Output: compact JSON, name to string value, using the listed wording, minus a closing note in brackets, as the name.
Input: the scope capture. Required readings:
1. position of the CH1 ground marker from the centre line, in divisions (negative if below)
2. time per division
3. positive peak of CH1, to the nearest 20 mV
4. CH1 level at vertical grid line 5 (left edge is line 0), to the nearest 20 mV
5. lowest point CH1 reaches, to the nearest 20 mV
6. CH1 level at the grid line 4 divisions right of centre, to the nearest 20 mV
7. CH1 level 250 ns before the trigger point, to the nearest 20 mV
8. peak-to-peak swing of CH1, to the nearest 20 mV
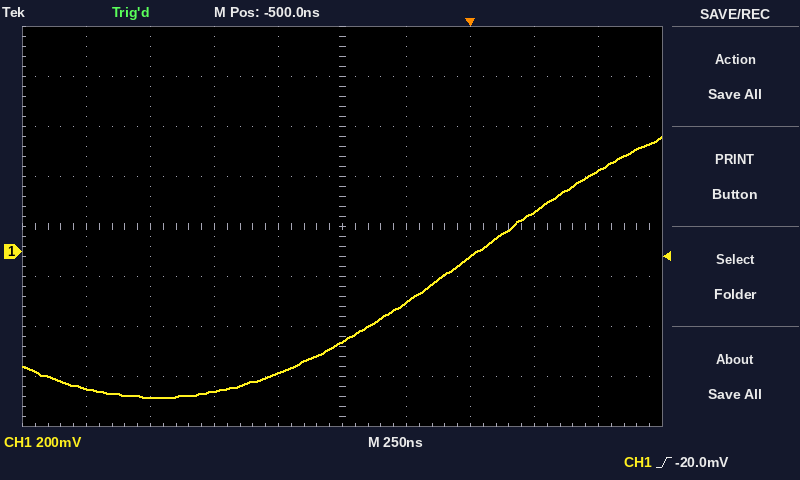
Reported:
{"position of the CH1 ground marker from the centre line, in divisions": "-0.5 div", "time per division": "250 ns", "positive peak of CH1, to the nearest 20 mV": "460 mV", "CH1 level at vertical grid line 5 (left edge is line 0), to the nearest 20 mV": "-360 mV", "lowest point CH1 reaches, to the nearest 20 mV": "-580 mV", "CH1 level at the grid line 4 divisions right of centre, to the nearest 20 mV": "320 mV", "CH1 level 250 ns before the trigger point, to the nearest 20 mV": "-200 mV", "peak-to-peak swing of CH1, to the nearest 20 mV": "1.04 V"}
